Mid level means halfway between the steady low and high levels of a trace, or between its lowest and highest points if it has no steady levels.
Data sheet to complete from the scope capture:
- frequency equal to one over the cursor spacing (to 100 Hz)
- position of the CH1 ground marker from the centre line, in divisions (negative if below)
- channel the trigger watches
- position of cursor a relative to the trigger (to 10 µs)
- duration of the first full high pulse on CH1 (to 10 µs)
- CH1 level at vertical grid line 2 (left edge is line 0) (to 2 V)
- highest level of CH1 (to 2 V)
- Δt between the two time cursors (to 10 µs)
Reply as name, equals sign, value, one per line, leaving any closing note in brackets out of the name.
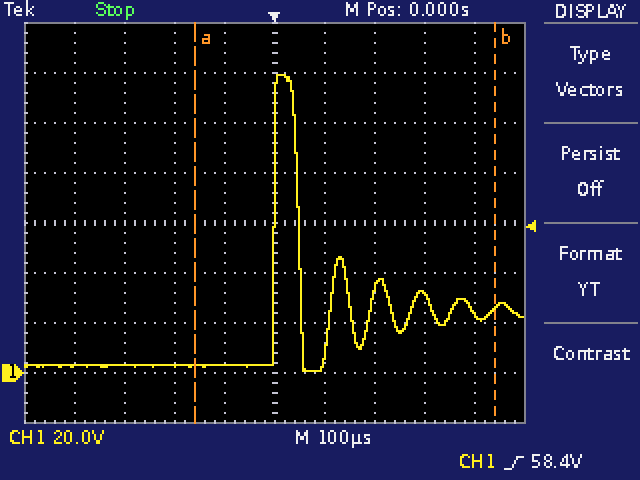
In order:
frequency equal to one over the cursor spacing = 1.7 kHz
position of the CH1 ground marker from the centre line, in divisions = -3.0 div
channel the trigger watches = CH1
position of cursor a relative to the trigger = -160 µs
duration of the first full high pulse on CH1 = 50 µs
CH1 level at vertical grid line 2 (left edge is line 0) = 4 V
highest level of CH1 = 120 V
Δt between the two time cursors = 600 µs
